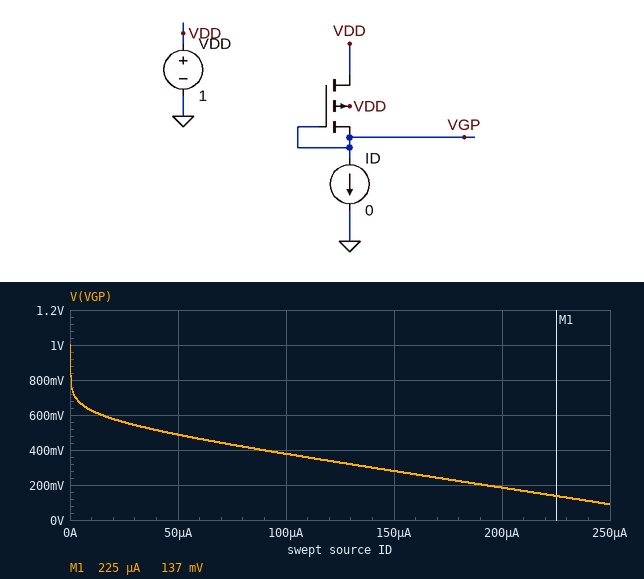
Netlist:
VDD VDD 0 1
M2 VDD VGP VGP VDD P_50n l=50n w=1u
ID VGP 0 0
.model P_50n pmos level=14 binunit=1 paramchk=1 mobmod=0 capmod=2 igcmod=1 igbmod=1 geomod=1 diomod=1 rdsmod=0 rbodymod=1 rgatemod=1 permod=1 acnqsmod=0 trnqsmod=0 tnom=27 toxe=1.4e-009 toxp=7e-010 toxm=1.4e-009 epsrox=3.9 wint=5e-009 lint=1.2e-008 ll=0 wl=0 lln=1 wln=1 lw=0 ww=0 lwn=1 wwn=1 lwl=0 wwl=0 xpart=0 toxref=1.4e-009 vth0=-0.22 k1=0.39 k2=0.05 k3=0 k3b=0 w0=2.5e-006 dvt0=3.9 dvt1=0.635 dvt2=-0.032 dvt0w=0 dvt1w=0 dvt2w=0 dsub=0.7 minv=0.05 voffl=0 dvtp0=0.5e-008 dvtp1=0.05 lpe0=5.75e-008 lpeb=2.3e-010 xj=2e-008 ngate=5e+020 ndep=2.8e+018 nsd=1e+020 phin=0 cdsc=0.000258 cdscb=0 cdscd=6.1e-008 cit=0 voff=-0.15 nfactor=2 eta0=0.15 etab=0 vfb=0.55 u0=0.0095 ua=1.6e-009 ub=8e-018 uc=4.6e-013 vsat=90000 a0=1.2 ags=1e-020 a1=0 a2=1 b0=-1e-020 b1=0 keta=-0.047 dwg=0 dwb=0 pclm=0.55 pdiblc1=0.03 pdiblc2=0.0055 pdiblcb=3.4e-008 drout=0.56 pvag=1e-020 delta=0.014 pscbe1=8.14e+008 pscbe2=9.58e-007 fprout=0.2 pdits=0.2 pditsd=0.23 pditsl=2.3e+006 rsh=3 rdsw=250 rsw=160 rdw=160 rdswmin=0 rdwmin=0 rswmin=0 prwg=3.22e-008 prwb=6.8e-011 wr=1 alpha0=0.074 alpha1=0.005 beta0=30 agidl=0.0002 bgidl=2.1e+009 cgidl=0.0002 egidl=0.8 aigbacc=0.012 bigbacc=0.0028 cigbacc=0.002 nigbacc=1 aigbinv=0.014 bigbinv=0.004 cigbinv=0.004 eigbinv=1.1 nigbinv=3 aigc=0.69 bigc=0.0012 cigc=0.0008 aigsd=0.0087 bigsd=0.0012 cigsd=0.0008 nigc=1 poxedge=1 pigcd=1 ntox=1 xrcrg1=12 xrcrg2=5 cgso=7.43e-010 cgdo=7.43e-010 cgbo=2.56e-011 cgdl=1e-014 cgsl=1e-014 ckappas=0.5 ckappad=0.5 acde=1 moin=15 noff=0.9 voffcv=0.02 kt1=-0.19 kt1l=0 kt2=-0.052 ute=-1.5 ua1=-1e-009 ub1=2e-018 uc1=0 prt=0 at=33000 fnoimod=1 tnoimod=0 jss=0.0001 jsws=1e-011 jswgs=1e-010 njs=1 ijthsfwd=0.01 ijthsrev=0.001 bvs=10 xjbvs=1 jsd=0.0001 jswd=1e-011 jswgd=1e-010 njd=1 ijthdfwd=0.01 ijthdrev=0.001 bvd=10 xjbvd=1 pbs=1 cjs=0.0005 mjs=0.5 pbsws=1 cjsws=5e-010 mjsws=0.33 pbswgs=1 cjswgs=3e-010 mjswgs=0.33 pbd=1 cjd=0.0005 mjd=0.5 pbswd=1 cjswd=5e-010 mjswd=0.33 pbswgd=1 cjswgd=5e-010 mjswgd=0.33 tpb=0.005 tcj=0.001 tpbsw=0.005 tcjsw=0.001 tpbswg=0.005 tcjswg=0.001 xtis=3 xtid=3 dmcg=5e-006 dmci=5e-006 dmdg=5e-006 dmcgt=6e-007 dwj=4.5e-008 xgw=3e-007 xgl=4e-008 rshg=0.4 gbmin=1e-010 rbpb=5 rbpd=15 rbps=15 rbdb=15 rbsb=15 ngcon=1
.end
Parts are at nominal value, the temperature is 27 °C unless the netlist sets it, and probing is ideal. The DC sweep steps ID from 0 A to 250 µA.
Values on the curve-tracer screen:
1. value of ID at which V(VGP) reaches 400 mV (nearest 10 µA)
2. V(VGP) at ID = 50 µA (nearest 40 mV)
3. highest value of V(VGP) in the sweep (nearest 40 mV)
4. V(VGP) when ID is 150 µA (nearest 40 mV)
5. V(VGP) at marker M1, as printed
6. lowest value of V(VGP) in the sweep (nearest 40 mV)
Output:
90 µA
480 mV
1.00 V
280 mV
137 mV
80 mV
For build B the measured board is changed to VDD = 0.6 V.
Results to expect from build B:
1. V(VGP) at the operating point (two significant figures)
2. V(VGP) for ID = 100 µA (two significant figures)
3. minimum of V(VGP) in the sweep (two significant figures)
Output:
600 mV
-22 mV
-310 mV
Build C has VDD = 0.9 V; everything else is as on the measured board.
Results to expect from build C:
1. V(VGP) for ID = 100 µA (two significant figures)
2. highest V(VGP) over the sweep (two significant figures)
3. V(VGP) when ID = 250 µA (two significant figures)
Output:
280 mV
900 mV
-10 mV
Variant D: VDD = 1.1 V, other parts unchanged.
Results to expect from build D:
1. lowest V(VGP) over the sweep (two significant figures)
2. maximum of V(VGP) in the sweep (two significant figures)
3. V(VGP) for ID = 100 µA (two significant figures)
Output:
190 mV
1.1 V
480 mV
